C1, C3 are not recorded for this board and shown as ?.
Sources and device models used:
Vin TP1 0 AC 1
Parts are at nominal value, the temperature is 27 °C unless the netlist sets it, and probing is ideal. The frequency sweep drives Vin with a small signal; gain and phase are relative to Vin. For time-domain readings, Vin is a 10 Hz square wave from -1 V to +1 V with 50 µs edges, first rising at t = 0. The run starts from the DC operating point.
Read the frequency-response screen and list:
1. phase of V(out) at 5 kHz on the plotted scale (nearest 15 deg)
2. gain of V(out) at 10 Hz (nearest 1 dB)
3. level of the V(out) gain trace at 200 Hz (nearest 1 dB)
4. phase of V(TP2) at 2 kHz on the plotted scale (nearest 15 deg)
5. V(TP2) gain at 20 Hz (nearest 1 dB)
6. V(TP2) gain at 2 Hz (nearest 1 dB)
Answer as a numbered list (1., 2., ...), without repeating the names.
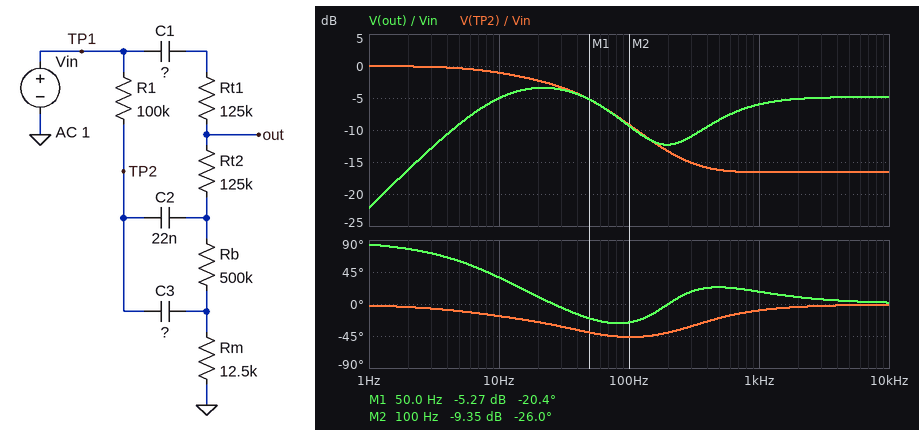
1. 0 deg
2. -5 dB
3. -12 dB
4. 0 deg
5. -2 dB
6. 0 dB
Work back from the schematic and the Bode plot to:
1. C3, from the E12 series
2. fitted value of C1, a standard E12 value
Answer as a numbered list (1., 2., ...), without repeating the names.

1. 39 nF
2. 1.2 nF
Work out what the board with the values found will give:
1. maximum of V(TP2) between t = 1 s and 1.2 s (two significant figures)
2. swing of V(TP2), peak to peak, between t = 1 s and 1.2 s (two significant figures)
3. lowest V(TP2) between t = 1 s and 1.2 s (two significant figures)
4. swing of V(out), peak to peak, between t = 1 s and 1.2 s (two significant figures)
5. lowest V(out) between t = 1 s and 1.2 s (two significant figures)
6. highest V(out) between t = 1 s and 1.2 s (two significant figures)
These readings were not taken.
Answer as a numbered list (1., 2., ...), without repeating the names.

1. 980 mV
2. 2.0 V
3. -980 mV
4. 2.0 V
5. -1.0 V
6. 1.0 V
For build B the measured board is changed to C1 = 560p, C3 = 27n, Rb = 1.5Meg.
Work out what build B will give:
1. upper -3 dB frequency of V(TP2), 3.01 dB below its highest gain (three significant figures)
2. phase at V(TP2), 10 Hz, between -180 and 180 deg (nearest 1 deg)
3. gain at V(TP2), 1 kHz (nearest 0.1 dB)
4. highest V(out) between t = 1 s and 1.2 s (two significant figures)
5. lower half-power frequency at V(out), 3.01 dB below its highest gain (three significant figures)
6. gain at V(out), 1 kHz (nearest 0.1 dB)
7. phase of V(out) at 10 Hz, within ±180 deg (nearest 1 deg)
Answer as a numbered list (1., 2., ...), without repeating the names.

1. 48.6 Hz
2. -10 deg
3. -17.0 dB
4. 1.2 V
5. 3.80 Hz
6. -8.6 dB
7. 15 deg
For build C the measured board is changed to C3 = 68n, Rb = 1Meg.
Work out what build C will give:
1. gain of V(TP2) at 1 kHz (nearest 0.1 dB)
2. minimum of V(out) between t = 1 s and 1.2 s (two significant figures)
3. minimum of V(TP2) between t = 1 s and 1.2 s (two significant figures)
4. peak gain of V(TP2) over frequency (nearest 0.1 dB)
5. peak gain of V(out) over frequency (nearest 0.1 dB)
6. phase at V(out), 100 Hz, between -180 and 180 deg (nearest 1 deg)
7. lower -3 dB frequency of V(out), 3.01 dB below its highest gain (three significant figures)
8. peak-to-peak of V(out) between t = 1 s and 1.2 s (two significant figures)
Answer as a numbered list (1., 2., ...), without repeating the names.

1. -16.9 dB
2. -950 mV
3. -960 mV
4. 0 dB
5. -2.7 dB
6. -21 deg
7. 4.18 Hz
8. 1.9 V
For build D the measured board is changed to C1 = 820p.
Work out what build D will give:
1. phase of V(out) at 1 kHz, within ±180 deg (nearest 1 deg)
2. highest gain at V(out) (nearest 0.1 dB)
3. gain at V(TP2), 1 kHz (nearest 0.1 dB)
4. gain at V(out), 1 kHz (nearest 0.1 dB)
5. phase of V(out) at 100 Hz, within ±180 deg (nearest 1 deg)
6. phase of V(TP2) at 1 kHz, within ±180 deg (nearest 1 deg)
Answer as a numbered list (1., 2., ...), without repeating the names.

1. 24 deg
2. -3.5 dB
3. -16.9 dB
4. -7.0 dB
5. -31 deg
6. -8 deg
